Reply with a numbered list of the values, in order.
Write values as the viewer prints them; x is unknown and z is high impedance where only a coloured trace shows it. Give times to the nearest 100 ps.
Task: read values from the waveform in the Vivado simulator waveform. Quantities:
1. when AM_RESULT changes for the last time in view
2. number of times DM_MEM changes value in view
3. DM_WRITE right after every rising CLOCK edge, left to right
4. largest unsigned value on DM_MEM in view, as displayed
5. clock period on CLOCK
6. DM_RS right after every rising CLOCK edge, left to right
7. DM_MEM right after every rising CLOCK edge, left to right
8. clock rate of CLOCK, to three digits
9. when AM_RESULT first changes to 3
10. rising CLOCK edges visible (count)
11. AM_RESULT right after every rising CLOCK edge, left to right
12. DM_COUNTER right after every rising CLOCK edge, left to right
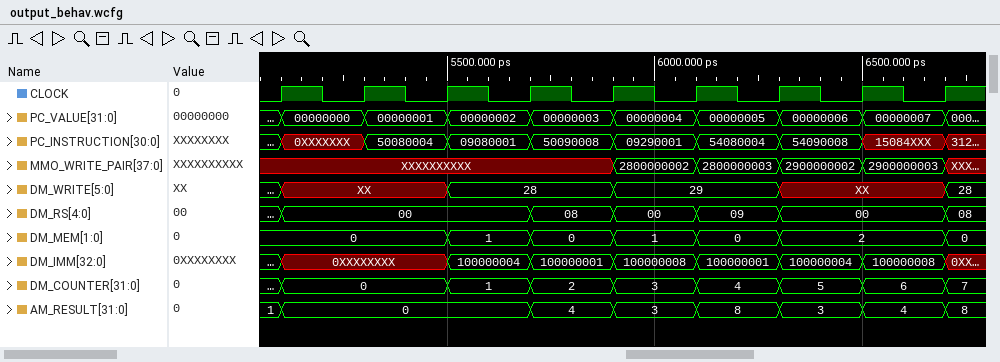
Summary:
1. 6700 ps
2. 6
3. XX, XX, 28, 28, 29, 29, XX, XX, 28
4. 2
5. 200 ps
6. 00, 00, 00, 08, 00, 09, 00, 00, 08
7. 0, 0, 1, 0, 1, 0, 2, 2, 0
8. 5.00 GHz
9. 5900 ps
10. 9
11. 0, 0, 0, 4, 3, 8, 3, 4, 8
12. 0, 0, 1, 2, 3, 4, 5, 6, 7
